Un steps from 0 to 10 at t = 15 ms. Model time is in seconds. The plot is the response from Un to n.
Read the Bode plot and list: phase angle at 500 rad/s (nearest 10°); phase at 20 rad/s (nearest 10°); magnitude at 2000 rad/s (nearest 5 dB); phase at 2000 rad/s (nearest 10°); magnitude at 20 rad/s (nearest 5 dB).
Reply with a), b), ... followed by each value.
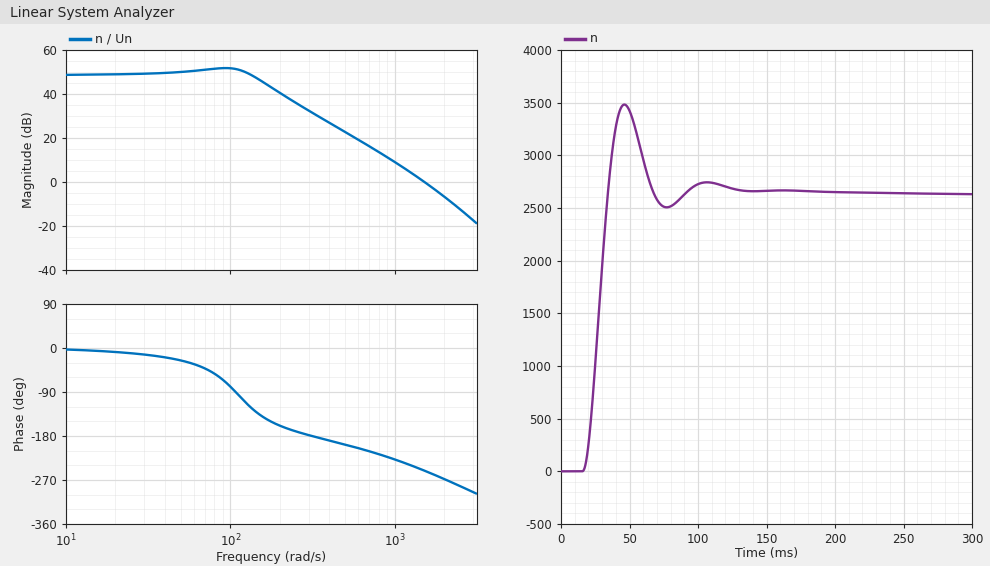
a) -200°
b) -10°
c) -5 dB
d) -270°
e) 50 dB
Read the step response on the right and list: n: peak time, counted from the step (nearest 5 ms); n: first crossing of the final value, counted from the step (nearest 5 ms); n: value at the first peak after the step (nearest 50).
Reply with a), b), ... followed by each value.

a) 30 ms
b) 20 ms
c) 3500
